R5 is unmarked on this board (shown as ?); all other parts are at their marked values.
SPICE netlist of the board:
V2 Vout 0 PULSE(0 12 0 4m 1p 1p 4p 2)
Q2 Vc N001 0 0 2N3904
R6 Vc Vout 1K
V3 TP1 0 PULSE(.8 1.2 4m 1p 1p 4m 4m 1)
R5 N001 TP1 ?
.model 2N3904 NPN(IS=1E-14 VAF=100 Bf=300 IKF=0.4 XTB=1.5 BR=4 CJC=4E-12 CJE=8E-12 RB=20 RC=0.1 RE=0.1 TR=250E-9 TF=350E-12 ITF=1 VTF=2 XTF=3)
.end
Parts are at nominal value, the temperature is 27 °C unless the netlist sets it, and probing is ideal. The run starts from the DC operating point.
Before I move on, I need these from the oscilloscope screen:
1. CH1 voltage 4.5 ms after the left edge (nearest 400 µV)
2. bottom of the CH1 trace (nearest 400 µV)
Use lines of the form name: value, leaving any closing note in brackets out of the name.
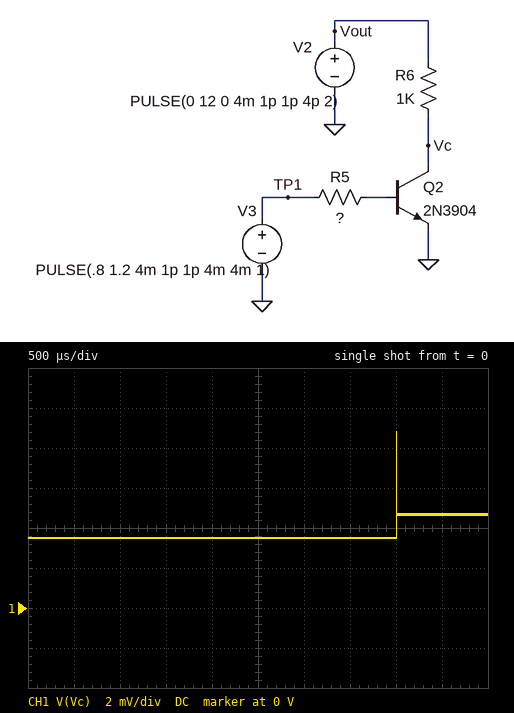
CH1 voltage 4.5 ms after the left edge: 4.8 mV
bottom of the CH1 trace: 3.6 mV
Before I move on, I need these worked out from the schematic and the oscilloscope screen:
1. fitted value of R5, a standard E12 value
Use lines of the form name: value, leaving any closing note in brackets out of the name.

fitted value of R5, a standard E12 value: 27 kΩ
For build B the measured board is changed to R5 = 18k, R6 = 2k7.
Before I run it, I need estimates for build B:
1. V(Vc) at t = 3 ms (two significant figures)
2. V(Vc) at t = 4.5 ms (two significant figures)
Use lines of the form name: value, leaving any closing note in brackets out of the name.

V(Vc) at t = 3 ms: 5.0 mV
V(Vc) at t = 4.5 ms: 5.5 mV
